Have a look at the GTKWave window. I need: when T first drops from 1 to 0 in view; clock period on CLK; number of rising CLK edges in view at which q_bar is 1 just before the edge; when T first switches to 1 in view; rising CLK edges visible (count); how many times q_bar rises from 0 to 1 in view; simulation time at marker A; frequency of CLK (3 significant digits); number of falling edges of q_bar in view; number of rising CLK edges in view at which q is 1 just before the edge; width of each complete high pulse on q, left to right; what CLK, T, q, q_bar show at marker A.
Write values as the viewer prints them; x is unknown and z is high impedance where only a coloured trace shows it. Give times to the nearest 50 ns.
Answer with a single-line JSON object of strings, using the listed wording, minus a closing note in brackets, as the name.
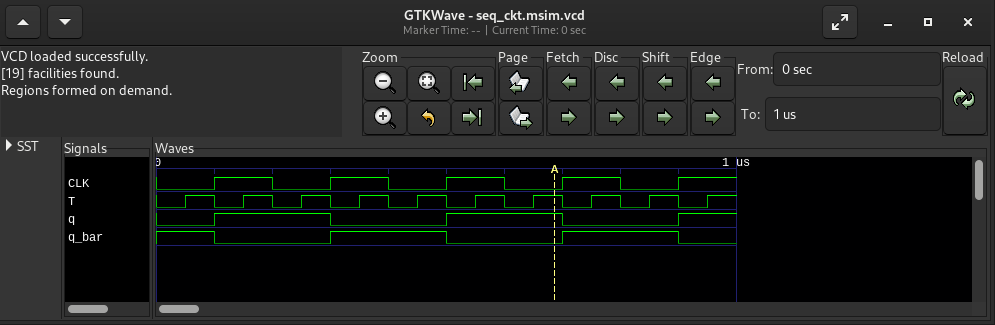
{"when T first drops from 1 to 0 in view": "100 ns", "clock period on CLK": "200 ns", "number of rising CLK edges in view at which q_bar is 1 just before the edge": "3", "when T first switches to 1 in view": "50 ns", "rising CLK edges visible": "5", "how many times q_bar rises from 0 to 1 in view": "2", "simulation time at marker A": "700 ns", "frequency of CLK": "5.00 MHz", "number of falling edges of q_bar in view": "3", "number of rising CLK edges in view at which q is 1 just before the edge": "2", "width of each complete high pulse on q, left to right": "200 ns, 200 ns", "what CLK, T, q, q_bar show at marker A": "CLK=0, T=1, q=1, q_bar=0"}
